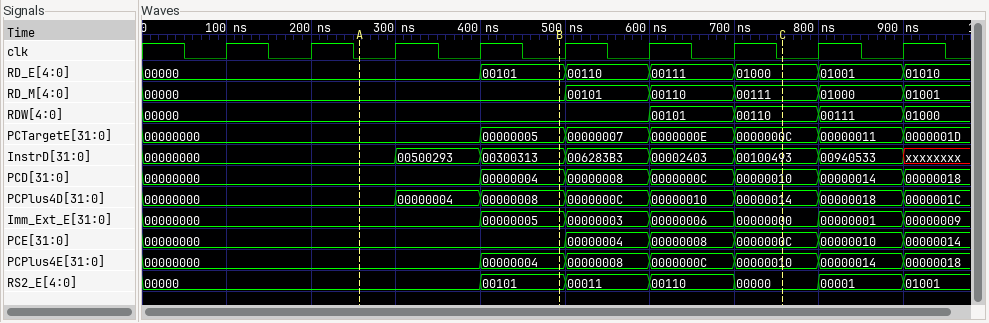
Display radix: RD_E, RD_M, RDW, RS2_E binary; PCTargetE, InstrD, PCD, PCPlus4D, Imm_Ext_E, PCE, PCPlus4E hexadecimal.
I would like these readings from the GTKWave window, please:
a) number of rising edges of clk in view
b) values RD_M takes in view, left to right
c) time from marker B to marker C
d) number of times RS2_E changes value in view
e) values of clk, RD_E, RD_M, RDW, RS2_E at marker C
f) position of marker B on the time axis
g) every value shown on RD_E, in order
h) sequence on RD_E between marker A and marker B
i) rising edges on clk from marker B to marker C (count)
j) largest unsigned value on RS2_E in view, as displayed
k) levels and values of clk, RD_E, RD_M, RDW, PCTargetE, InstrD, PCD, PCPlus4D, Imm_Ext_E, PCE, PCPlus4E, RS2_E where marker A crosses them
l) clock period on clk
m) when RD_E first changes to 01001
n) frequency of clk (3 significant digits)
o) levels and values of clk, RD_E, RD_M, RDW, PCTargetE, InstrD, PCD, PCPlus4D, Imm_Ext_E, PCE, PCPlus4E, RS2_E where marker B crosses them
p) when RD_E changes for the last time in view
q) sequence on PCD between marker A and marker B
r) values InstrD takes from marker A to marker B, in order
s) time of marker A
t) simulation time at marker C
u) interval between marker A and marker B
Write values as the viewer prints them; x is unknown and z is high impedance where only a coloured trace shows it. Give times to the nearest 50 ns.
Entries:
9
00000, 00101, 00110, 00111, 01000, 01001
250 ns
6
clk=0, RD_E=01000, RD_M=00111, RDW=00110, RS2_E=00000
500 ns
00000, 00101, 00110, 00111, 01000, 01001, 01010
00000, 00101
3
01001
clk=0, RD_E=00000, RD_M=00000, RDW=00000, PCTargetE=00000000, InstrD=00000000, PCD=00000000, PCPlus4D=00000000, Imm_Ext_E=00000000, PCE=00000000, PCPlus4E=00000000, RS2_E=00000
100 ns
800 ns
10.0 MHz
clk=0, RD_E=00101, RD_M=00000, RDW=00000, PCTargetE=00000005, InstrD=00300313, PCD=00000004, PCPlus4D=00000008, Imm_Ext_E=00000005, PCE=00000000, PCPlus4E=00000004, RS2_E=00101
900 ns
00000000, 00000004
00000000, 00500293, 00300313
250 ns
750 ns
250 ns
